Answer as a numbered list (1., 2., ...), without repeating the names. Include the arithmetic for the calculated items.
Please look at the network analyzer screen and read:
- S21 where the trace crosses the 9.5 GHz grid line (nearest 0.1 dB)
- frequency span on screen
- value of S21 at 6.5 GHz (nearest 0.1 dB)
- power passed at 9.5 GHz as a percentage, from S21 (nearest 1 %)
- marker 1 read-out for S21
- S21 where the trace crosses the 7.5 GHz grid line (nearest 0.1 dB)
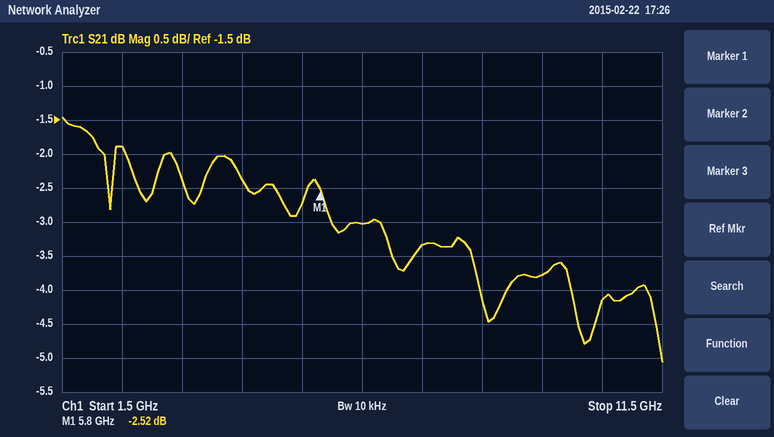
1. -3.8 dB
2. 10 GHz
3. -3.0 dB
4. 10^(-3.8/10) ≈ 42 %
5. -2.52 dB
6. -3.3 dB
